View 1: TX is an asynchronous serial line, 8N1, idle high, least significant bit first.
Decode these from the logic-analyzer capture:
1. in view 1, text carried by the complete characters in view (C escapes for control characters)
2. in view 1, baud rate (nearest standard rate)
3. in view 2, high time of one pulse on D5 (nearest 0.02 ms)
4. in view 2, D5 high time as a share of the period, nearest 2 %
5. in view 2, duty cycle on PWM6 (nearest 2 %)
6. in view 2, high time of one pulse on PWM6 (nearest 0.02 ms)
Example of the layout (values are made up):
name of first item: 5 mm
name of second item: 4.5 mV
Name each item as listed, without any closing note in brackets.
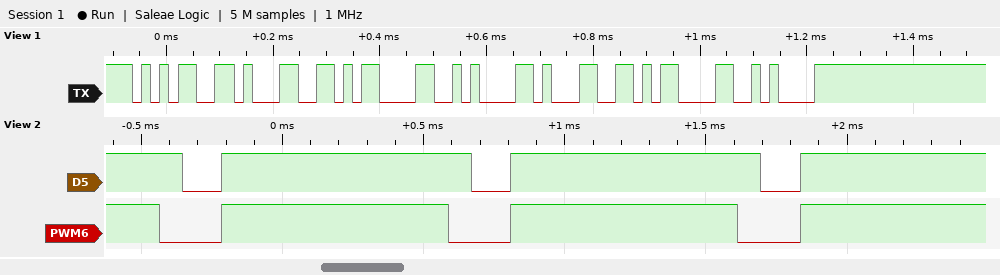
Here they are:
in view 1, text carried by the complete characters in view: "51\r\n1\r\n"
in view 1, baud rate: 57600 baud
in view 2, high time of one pulse on D5: 0.88 ms
in view 2, D5 high time as a share of the period, nearest 2 %: 86 %
in view 2, duty cycle on PWM6: 78 %
in view 2, high time of one pulse on PWM6: 0.80 ms
